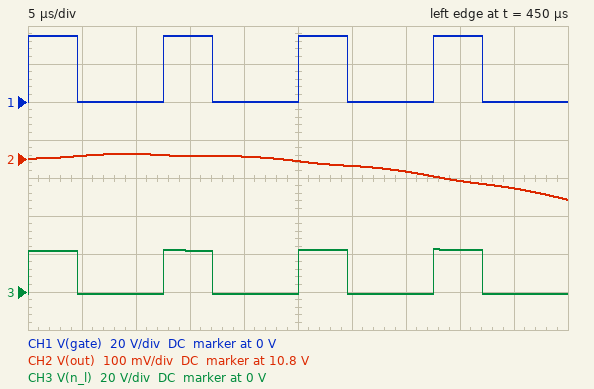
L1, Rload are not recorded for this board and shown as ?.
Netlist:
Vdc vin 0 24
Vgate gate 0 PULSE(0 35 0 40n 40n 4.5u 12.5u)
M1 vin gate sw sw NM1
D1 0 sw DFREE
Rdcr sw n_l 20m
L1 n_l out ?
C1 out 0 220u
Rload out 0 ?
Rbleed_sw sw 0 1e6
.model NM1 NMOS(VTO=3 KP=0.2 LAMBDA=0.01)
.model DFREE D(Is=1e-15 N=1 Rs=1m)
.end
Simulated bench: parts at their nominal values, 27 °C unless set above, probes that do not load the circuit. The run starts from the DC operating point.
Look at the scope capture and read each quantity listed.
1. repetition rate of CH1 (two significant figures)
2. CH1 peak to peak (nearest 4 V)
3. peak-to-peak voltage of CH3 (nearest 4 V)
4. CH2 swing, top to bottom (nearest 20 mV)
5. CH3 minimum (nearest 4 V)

80 kHz
36 V
24 V
120 mV
0 V
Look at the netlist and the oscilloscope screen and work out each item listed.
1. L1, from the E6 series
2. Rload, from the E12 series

100 µH
2.7 Ω
